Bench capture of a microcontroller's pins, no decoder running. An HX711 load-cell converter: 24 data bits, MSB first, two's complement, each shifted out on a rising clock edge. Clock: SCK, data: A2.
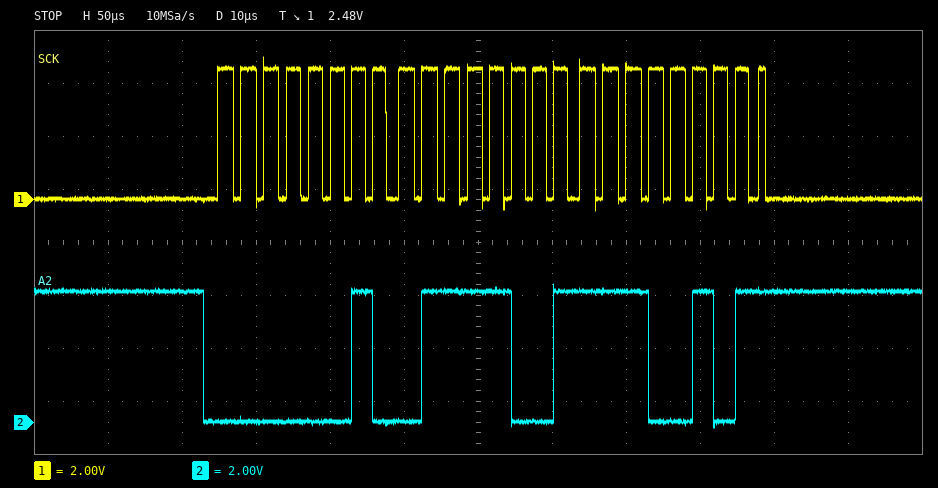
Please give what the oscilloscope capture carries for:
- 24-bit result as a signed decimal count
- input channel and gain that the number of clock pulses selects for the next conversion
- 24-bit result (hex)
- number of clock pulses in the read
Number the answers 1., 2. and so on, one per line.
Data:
1. 162277
2. channel A, gain 128
3. 0x0279E5
4. 25
